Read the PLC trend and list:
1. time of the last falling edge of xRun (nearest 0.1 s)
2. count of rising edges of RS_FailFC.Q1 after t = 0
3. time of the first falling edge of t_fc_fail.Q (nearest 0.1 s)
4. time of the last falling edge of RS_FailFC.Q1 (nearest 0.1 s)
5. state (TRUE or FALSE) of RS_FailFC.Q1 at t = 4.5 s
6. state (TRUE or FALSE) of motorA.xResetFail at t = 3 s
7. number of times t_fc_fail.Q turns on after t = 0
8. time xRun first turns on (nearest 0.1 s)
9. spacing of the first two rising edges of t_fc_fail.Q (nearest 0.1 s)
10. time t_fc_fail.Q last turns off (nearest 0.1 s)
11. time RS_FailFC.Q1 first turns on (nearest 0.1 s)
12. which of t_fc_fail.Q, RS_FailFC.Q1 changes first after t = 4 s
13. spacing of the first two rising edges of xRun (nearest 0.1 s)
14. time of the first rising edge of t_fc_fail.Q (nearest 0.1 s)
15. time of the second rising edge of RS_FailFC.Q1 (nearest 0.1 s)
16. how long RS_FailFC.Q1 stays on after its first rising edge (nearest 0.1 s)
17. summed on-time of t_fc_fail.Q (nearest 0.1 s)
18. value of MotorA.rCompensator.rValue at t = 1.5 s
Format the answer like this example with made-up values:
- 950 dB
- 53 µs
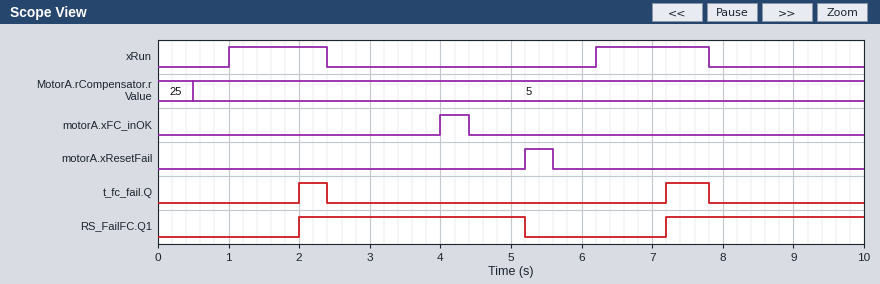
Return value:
- 7.8 s
- 2
- 2.4 s
- 5.2 s
- TRUE
- FALSE
- 2
- 1.0 s
- 5.2 s
- 7.8 s
- 2.0 s
- RS_FailFC.Q1
- 5.2 s
- 2.0 s
- 7.2 s
- 3.2 s
- 1.0 s
- 5
